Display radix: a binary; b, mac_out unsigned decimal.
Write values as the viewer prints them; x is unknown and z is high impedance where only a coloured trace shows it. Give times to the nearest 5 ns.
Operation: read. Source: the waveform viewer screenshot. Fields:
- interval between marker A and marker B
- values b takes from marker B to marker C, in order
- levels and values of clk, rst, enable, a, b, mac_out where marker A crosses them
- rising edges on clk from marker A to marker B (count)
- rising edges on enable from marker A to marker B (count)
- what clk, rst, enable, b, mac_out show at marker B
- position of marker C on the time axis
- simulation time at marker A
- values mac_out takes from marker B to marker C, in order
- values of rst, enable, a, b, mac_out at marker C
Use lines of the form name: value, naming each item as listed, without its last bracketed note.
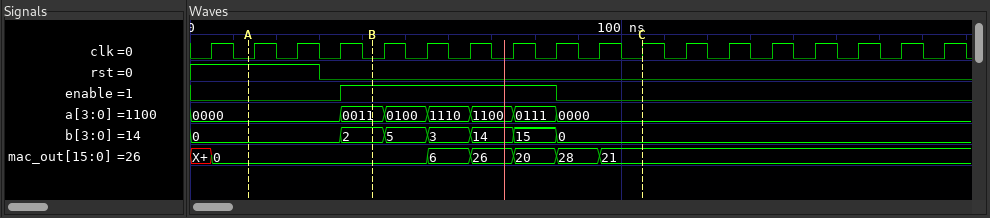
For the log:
interval between marker A and marker B: 30 ns
values b takes from marker B to marker C, in order: 2, 5, 3, 14, 15, 0
levels and values of clk, rst, enable, a, b, mac_out where marker A crosses them: clk=0, rst=1, enable=0, a=0000, b=0, mac_out=0
rising edges on clk from marker A to marker B: 3
rising edges on enable from marker A to marker B: 1
what clk, rst, enable, b, mac_out show at marker B: clk=0, rst=0, enable=1, b=2, mac_out=0
position of marker C on the time axis: 105 ns
simulation time at marker A: 15 ns
values mac_out takes from marker B to marker C, in order: 0, 6, 26, 20, 28, 21
values of rst, enable, a, b, mac_out at marker C: rst=0, enable=0, a=0000, b=0, mac_out=21
